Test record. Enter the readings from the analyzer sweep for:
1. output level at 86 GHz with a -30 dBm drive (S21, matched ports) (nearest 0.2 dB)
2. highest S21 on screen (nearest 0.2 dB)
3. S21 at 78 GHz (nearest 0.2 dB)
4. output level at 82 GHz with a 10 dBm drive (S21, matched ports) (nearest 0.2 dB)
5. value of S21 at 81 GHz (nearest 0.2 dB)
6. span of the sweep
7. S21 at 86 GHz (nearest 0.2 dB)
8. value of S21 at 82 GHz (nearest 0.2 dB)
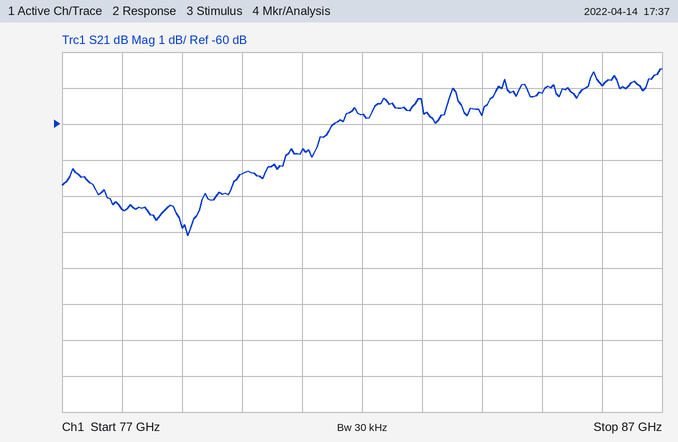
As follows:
-89.0 dBm
-58.4 dB
-62.4 dB
-49.8 dBm
-60.8 dB
10 GHz
-59.0 dB
-59.8 dB
